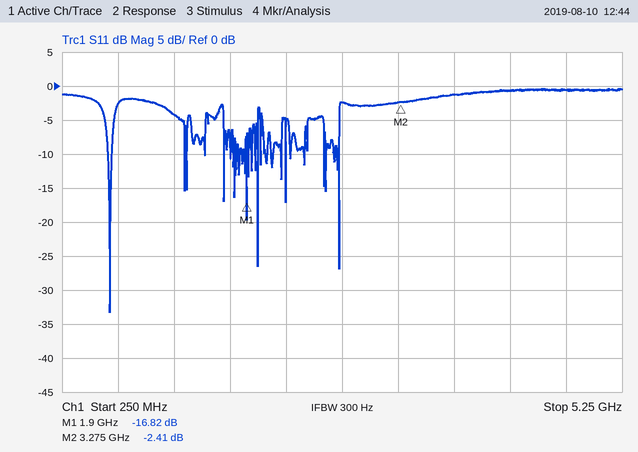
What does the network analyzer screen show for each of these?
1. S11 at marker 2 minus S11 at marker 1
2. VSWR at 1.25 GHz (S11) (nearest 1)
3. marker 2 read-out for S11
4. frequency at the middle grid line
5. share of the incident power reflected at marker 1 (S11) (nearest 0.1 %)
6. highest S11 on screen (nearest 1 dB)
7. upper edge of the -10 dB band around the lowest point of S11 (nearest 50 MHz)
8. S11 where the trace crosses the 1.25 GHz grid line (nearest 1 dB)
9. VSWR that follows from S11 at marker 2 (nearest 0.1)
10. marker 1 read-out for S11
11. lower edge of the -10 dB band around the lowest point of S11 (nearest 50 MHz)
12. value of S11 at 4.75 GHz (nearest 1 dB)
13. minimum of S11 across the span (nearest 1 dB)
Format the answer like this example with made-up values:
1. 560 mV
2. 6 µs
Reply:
1. 14.41 dB
2. 4
3. -2.41 dB
4. 2.75 GHz
5. 2.1 %
6. 0 dB
7. 700 MHz
8. -4 dB
9. 7.3
10. -16.82 dB
11. 650 MHz
12. -1 dB
13. -33 dB
